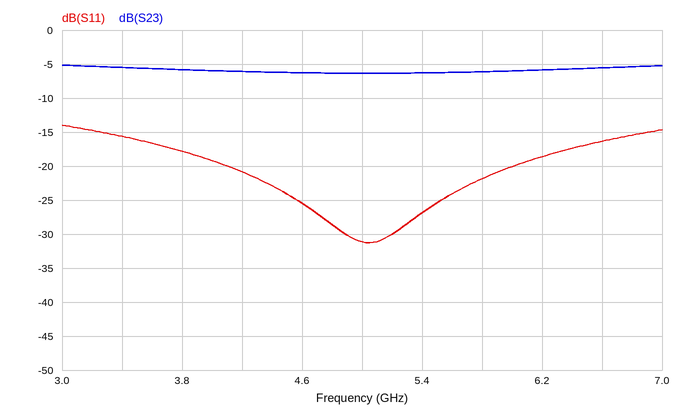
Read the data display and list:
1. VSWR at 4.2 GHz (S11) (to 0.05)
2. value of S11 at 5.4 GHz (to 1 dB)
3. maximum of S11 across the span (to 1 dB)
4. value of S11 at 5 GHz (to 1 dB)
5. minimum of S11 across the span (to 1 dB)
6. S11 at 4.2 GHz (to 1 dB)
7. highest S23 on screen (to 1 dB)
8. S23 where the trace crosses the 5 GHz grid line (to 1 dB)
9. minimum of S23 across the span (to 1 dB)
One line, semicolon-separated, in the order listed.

1.20; -27 dB; -14 dB; -31 dB; -31 dB; -21 dB; -5 dB; -6 dB; -6 dB
